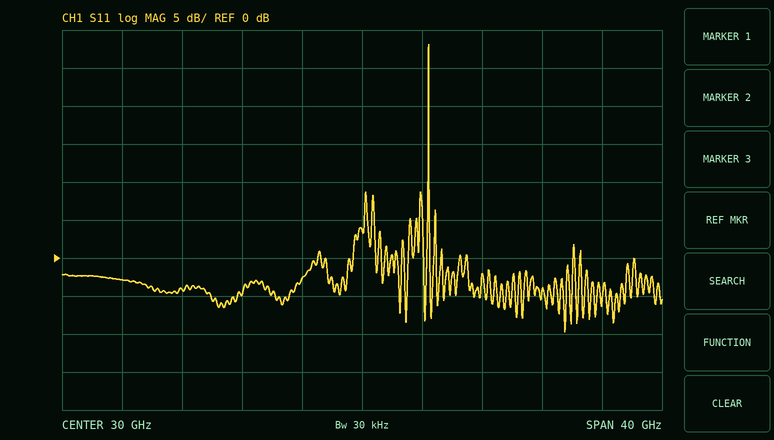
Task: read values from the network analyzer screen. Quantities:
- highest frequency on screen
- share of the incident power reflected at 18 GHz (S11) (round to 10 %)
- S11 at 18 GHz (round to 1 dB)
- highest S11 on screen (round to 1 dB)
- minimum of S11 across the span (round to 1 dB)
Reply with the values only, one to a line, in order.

50 GHz
40 %
-4 dB
28 dB
-10 dB
